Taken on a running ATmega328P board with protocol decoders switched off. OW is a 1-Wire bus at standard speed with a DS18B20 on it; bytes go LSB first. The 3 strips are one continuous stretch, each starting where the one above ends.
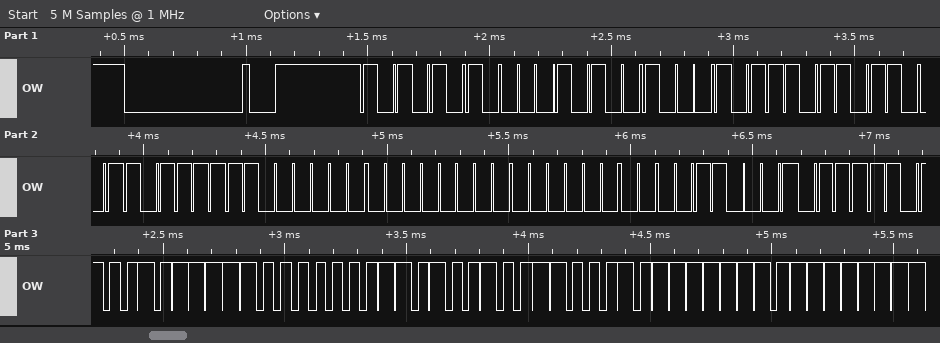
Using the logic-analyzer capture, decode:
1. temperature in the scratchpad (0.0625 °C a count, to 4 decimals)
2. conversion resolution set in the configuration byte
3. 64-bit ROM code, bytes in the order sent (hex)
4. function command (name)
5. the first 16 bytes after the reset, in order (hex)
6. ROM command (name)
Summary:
31.2500 °C
12 bits
28 D1 6D F6 03 00 00 8C
Read Scratchpad
55 28 D1 6D F6 03 00 00 8C BE F4 01 4B 46 7F FF
Match ROM
